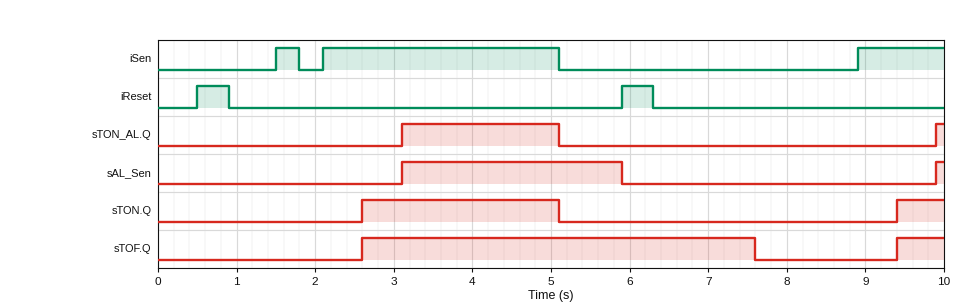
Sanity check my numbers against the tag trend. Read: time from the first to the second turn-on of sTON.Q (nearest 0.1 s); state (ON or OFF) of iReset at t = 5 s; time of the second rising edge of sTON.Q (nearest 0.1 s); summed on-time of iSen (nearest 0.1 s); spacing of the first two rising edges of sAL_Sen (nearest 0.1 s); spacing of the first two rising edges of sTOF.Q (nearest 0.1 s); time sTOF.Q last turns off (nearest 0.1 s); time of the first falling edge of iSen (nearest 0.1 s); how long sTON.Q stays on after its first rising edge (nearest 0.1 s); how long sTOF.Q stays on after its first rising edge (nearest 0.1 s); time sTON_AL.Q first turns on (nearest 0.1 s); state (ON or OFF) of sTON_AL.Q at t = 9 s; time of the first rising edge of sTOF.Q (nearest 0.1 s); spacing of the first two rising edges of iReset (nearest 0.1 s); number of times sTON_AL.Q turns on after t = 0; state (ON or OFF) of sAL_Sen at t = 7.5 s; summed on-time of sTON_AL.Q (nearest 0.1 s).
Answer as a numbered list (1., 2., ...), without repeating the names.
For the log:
1. 6.8 s
2. OFF
3. 9.4 s
4. 4.4 s
5. 6.8 s
6. 6.8 s
7. 7.6 s
8. 1.8 s
9. 2.5 s
10. 5.0 s
11. 3.1 s
12. OFF
13. 2.6 s
14. 5.4 s
15. 2
16. OFF
17. 2.1 s
